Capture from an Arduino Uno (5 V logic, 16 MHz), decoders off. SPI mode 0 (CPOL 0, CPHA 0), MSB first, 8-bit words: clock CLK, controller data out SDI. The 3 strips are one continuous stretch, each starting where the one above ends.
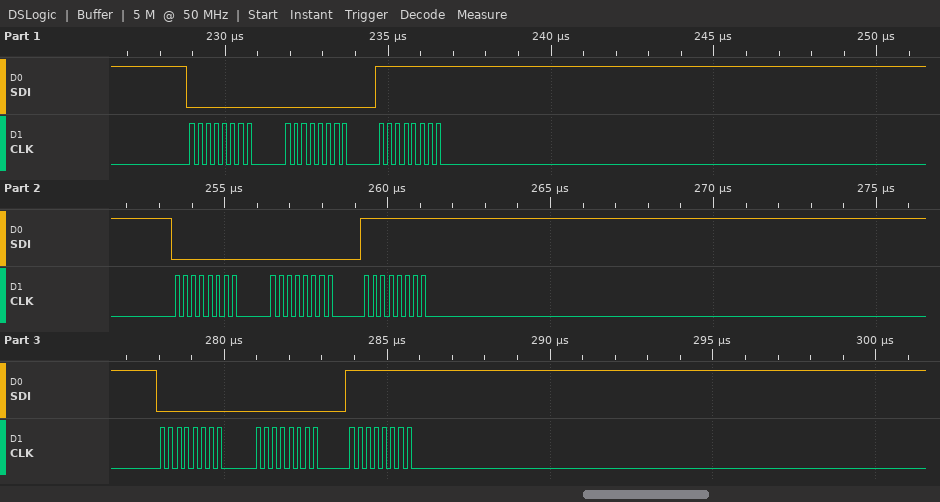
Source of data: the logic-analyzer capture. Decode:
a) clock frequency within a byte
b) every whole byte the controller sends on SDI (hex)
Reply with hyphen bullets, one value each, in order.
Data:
- 4 MHz
- 00 00 FF 00 00 FF 00 00 FF
